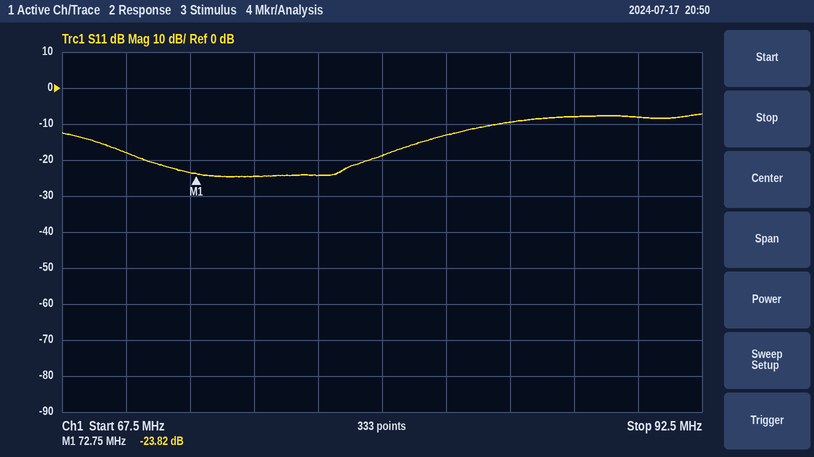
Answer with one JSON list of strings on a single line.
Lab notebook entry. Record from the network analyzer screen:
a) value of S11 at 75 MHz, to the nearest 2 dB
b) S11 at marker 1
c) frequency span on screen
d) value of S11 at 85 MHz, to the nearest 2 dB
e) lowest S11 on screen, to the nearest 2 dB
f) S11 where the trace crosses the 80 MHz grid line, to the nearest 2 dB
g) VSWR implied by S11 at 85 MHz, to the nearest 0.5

["-24 dB", "-23.82 dB", "25 MHz", "-10 dB", "-24 dB", "-18 dB", "2.0"]
